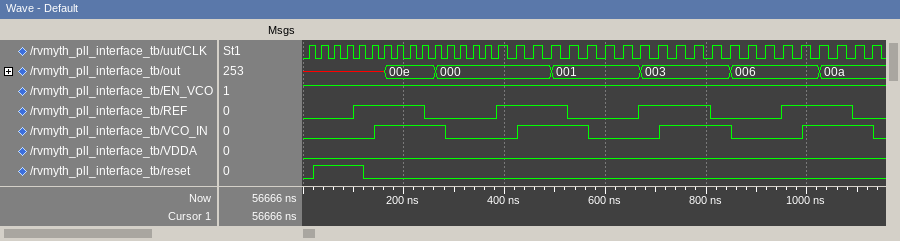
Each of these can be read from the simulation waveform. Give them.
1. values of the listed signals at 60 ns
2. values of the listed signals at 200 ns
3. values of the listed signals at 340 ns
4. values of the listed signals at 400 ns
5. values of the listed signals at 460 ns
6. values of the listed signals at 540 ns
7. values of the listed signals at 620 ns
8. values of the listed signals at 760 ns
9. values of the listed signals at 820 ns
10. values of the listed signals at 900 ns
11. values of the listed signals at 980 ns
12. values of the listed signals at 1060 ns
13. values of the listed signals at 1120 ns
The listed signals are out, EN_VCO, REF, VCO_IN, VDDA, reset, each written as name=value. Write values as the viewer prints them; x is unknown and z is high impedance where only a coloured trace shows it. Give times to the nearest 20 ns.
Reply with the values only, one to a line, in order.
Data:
out=x, EN_VCO=1, REF=0, VCO_IN=0, VDDA=0, reset=1
out=00e, EN_VCO=1, REF=1, VCO_IN=1, VDDA=0, reset=0
out=000, EN_VCO=1, REF=0, VCO_IN=0, VDDA=0, reset=0
out=000, EN_VCO=1, REF=1, VCO_IN=0, VDDA=0, reset=0
out=000, EN_VCO=1, REF=1, VCO_IN=1, VDDA=0, reset=0
out=001, EN_VCO=1, REF=0, VCO_IN=1, VDDA=0, reset=0
out=001, EN_VCO=1, REF=0, VCO_IN=0, VDDA=0, reset=0
out=003, EN_VCO=1, REF=1, VCO_IN=1, VDDA=0, reset=0
out=003, EN_VCO=1, REF=0, VCO_IN=1, VDDA=0, reset=0
out=006, EN_VCO=1, REF=0, VCO_IN=0, VDDA=0, reset=0
out=006, EN_VCO=1, REF=1, VCO_IN=0, VDDA=0, reset=0
out=00a, EN_VCO=1, REF=1, VCO_IN=1, VDDA=0, reset=0
out=00a, EN_VCO=1, REF=0, VCO_IN=1, VDDA=0, reset=0
